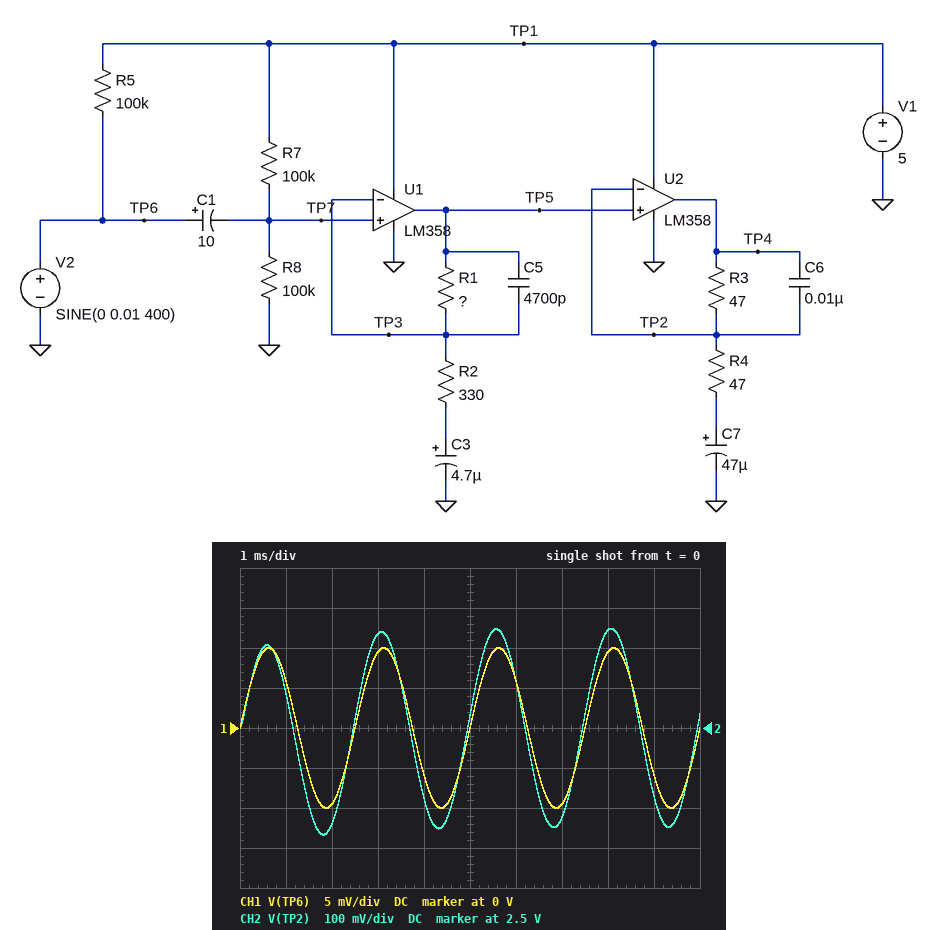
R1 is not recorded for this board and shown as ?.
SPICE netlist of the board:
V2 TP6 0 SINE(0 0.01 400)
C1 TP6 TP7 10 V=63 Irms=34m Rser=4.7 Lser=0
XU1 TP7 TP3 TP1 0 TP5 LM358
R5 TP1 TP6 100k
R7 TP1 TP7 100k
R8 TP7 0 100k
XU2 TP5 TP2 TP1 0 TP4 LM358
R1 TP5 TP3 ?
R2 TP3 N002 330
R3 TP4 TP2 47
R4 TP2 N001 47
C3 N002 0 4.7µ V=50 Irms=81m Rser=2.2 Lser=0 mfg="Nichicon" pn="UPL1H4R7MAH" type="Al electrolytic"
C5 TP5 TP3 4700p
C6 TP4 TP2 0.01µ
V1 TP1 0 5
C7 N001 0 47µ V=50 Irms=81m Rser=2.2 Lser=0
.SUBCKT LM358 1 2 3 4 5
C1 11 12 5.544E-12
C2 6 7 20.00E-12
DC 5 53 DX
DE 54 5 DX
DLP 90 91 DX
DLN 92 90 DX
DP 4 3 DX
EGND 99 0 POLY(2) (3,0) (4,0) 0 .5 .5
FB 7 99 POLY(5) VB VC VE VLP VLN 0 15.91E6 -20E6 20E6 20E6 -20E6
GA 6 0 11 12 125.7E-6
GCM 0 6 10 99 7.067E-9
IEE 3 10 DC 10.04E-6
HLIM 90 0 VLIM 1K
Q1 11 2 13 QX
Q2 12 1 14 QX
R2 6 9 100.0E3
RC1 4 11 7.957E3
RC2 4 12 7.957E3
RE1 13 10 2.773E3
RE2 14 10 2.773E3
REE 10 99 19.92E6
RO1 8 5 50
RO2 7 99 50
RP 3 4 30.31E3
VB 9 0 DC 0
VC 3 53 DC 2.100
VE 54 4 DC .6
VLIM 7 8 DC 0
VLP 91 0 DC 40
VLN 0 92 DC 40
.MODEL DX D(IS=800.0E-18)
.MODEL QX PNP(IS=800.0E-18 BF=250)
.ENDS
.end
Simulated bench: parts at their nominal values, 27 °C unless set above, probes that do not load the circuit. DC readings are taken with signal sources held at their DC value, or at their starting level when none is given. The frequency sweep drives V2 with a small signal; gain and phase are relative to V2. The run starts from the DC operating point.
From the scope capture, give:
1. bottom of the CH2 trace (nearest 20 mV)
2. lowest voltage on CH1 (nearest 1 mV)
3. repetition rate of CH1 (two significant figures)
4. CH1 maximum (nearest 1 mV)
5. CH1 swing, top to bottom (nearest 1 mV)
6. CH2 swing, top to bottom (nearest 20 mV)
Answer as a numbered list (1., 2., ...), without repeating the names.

1. 2.24 V
2. -10 mV
3. 400 Hz
4. 10 mV
5. 20 mV
6. 520 mV
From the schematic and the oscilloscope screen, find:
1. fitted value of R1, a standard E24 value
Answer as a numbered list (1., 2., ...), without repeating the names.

1. 8.2 kΩ
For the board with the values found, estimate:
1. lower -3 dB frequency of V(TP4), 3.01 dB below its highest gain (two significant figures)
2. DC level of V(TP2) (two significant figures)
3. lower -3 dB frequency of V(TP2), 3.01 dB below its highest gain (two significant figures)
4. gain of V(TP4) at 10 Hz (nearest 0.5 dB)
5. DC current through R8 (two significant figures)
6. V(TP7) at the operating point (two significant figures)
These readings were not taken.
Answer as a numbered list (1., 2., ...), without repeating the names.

1. 120 Hz
2. 2.5 V
3. 97 Hz
4. 9.0 dB
5. 25 µA
6. 2.5 V
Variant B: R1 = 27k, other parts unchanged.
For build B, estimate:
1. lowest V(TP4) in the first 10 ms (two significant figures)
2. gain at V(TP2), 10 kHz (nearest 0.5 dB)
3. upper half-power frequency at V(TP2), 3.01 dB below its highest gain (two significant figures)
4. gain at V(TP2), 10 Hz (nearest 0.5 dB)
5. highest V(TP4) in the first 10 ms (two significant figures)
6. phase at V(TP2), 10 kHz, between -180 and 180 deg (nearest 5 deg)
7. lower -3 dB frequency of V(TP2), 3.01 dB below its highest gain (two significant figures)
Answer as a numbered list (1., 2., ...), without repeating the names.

1. 910 mV
2. 19.5 dB
3. 1.3 kHz
4. 18.0 dB
5. 3.5 V
6. -80 deg
7. 88 Hz
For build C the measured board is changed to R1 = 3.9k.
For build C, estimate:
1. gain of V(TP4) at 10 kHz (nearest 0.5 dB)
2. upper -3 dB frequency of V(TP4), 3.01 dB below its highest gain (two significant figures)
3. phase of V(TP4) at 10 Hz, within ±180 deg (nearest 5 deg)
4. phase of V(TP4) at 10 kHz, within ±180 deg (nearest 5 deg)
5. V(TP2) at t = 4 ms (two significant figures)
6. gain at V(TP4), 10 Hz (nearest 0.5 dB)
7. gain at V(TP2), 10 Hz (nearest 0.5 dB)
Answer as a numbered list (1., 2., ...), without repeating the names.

1. 24.0 dB
2. 8.1 kHz
3. 55 deg
4. -50 deg
5. 2.4 V
6. 4.5 dB
7. 4.0 dB
